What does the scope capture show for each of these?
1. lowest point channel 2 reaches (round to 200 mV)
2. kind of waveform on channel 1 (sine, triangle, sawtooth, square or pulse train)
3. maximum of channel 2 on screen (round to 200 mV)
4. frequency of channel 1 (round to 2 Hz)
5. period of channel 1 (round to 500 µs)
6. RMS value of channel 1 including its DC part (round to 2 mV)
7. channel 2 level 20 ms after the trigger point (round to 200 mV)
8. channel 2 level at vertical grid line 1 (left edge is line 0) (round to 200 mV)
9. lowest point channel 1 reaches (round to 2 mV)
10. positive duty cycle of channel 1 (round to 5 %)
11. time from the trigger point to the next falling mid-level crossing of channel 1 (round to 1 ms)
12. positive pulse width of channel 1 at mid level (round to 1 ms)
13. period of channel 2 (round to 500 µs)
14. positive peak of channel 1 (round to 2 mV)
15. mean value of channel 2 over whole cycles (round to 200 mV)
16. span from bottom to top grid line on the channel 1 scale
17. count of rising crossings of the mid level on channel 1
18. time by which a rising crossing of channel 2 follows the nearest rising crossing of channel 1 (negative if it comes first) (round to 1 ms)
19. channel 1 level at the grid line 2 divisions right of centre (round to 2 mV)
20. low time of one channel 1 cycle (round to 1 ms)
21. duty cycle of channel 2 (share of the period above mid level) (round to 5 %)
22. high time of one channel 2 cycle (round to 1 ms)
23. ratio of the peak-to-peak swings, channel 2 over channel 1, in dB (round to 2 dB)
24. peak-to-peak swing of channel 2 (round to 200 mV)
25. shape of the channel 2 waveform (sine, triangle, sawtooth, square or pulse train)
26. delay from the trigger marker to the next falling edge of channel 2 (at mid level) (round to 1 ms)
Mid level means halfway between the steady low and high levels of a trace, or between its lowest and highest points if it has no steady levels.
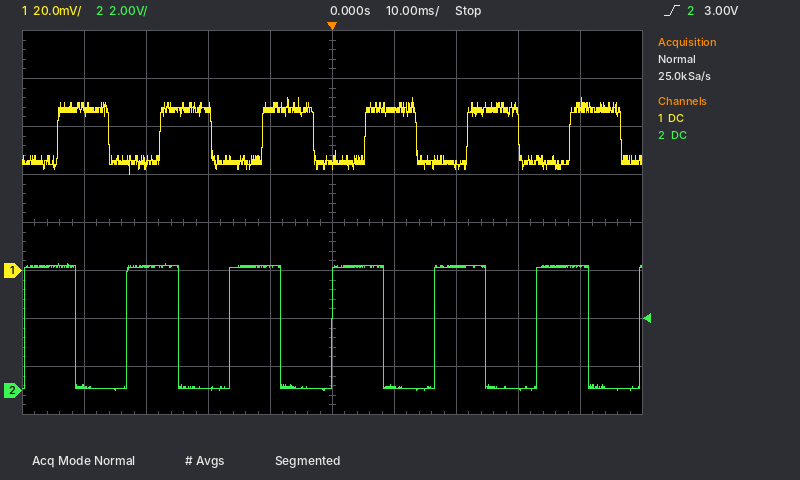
0.0 V
square
5.2 V
60 Hz
16.5 ms
58 mV
5.2 V
200 mV
40 mV
50 %
14 ms
8 ms
16.5 ms
72 mV
2.6 V
160 mV
6
-5 ms
44 mV
8 ms
50 %
8 ms
44 dB
5.2 V
square
8 ms
